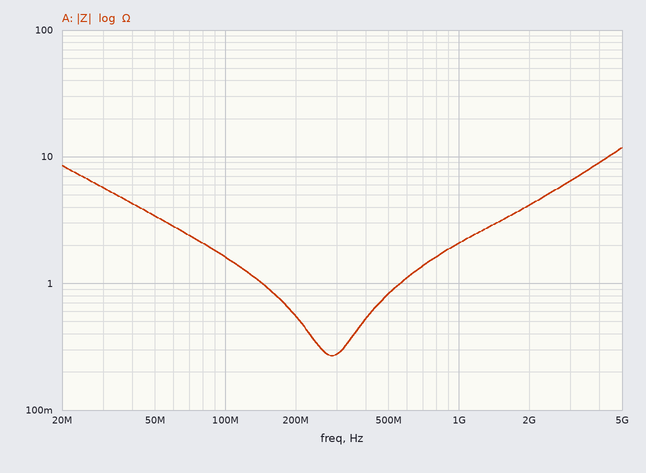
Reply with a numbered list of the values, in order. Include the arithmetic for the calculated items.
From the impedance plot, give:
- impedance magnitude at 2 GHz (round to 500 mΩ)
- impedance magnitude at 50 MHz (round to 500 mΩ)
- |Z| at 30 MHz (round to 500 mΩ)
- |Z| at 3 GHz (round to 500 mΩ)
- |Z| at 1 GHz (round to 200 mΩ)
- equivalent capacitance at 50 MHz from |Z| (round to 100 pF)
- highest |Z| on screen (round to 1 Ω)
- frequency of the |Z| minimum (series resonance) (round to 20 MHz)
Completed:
1. 4.0 Ω
2. 3.5 Ω
3. 5.5 Ω
4. 6.5 Ω
5. 2.0 Ω
6. C = 1/(2π × 50 MHz × 3.5 Ω) ≈ 909 pF, so 900 pF to the nearest 100 pF
7. 12 Ω
8. 280 MHz
